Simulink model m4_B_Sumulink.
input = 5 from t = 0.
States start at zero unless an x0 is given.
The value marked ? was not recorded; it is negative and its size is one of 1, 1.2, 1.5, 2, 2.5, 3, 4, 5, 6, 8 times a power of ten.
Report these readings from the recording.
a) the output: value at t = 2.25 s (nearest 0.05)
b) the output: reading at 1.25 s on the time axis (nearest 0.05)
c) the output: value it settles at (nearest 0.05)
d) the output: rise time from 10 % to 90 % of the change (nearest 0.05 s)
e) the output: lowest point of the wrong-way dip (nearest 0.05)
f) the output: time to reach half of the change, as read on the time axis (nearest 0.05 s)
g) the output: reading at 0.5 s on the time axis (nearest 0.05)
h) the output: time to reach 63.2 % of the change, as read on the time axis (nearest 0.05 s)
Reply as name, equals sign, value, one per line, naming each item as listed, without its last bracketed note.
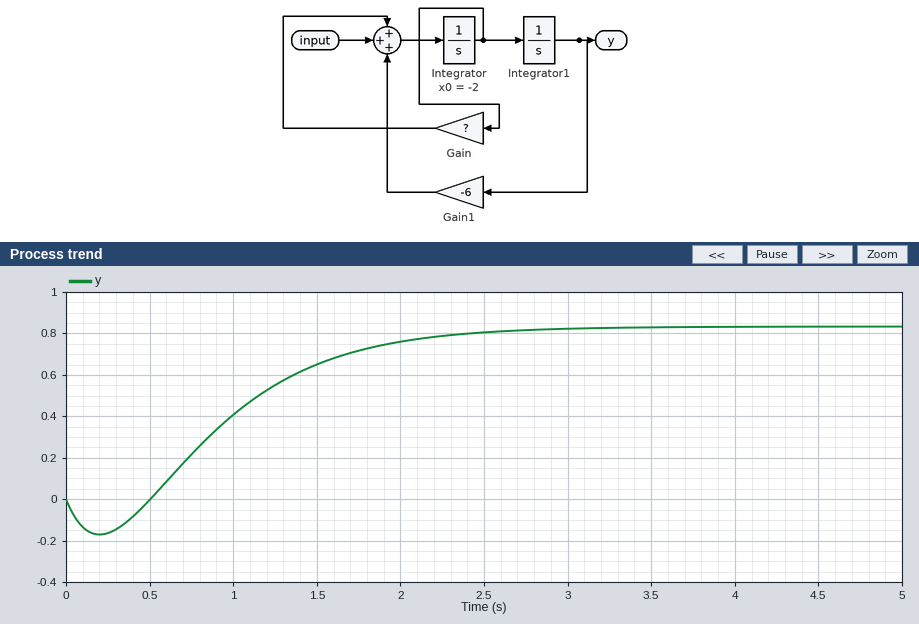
the output: value at t = 2.25 s = 0.80
the output: reading at 1.25 s on the time axis = 0.55
the output: value it settles at = 0.85
the output: rise time from 10 % to 90 % of the change = 1.35 s
the output: lowest point of the wrong-way dip = -0.15
the output: time to reach half of the change, as read on the time axis = 1.00 s
the output: reading at 0.5 s on the time axis = 0.00
the output: time to reach 63.2 % of the change, as read on the time axis = 1.20 s
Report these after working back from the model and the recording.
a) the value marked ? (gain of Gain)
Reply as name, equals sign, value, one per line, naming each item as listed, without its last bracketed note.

the value marked ? = -5
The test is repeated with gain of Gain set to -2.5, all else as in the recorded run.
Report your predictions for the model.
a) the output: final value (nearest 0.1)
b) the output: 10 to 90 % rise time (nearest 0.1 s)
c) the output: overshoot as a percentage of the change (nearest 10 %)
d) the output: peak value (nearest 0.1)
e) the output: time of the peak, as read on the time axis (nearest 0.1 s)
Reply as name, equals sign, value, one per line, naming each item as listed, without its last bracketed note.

the output: final value = 0.8
the output: 10 to 90 % rise time = 0.5 s
the output: overshoot as a percentage of the change = 20 %
the output: peak value = 1.0
the output: time of the peak, as read on the time axis = 1.7 s
